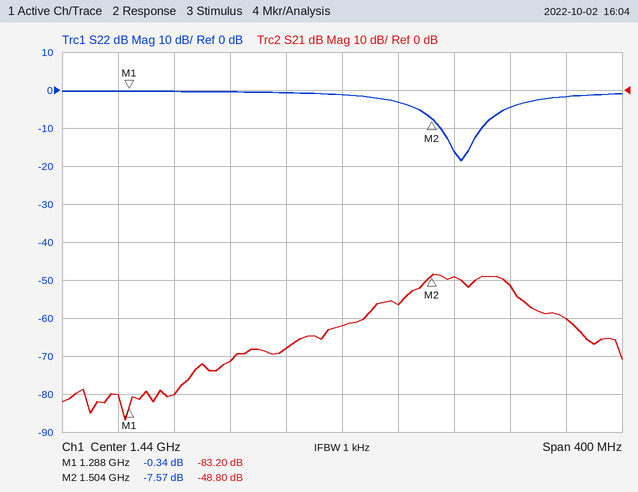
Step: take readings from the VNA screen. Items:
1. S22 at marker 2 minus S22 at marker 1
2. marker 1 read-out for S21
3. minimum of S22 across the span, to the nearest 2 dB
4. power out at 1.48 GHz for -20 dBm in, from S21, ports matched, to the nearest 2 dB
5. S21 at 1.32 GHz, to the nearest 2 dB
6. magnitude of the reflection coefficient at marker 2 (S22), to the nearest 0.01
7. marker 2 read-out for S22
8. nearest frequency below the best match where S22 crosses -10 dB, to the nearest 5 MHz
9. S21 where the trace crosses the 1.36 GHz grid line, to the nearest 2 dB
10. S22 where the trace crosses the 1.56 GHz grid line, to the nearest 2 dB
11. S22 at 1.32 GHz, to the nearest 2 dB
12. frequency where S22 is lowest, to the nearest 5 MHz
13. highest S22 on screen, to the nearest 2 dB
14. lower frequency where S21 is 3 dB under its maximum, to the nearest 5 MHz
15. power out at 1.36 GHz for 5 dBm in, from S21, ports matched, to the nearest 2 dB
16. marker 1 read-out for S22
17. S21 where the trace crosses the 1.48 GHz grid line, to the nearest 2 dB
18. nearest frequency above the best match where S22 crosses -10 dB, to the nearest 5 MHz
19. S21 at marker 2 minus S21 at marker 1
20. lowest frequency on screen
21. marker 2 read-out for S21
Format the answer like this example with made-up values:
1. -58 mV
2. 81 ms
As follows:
1. -7.23 dB
2. -83.20 dB
3. -18 dB
4. -76 dBm
5. -80 dB
6. 0.42
7. -7.57 dB
8. 1.510 GHz
9. -72 dB
10. -4 dB
11. 0 dB
12. 1.525 GHz
13. 0 dB
14. 1.495 GHz
15. -66 dBm
16. -0.34 dB
17. -56 dB
18. 1.540 GHz
19. 34.40 dB
20. 1.24 GHz
21. -48.80 dB
